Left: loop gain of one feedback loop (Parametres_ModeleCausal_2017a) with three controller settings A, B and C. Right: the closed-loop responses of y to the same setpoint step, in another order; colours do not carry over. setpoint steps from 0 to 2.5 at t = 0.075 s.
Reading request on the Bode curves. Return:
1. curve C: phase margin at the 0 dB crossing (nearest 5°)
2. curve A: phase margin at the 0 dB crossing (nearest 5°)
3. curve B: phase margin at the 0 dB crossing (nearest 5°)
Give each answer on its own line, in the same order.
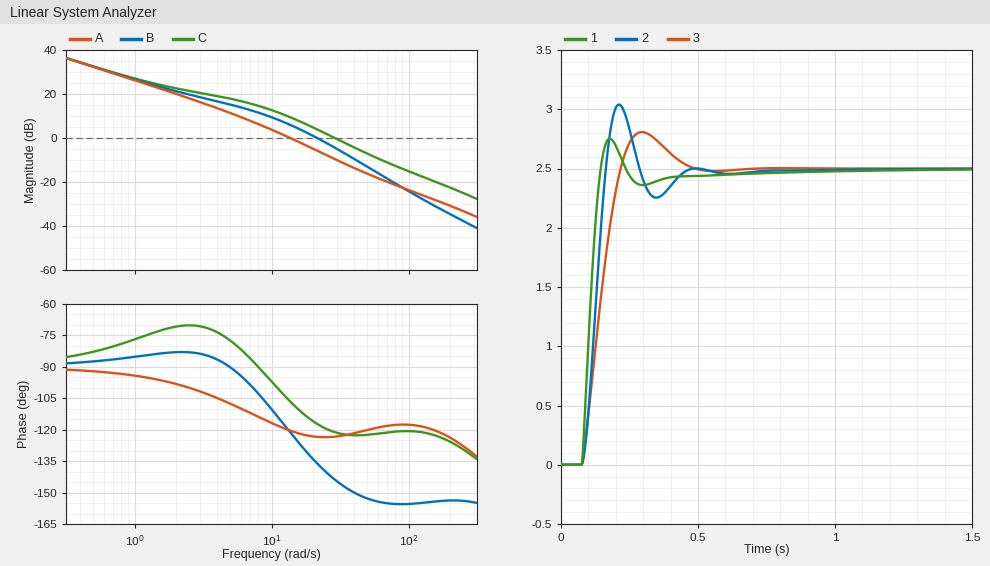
60°
60°
45°
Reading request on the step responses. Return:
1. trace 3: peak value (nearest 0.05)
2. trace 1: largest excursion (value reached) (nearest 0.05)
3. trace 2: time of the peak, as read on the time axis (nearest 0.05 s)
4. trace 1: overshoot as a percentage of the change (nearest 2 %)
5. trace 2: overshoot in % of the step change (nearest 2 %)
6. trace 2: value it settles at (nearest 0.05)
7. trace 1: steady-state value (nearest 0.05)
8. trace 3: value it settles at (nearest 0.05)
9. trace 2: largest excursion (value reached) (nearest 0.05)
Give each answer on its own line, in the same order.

2.80
2.75
0.20 s
10 %
22 %
2.50
2.50
2.50
3.05
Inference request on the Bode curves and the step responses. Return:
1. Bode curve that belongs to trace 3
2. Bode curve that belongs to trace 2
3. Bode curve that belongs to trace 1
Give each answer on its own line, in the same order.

A
B
C
